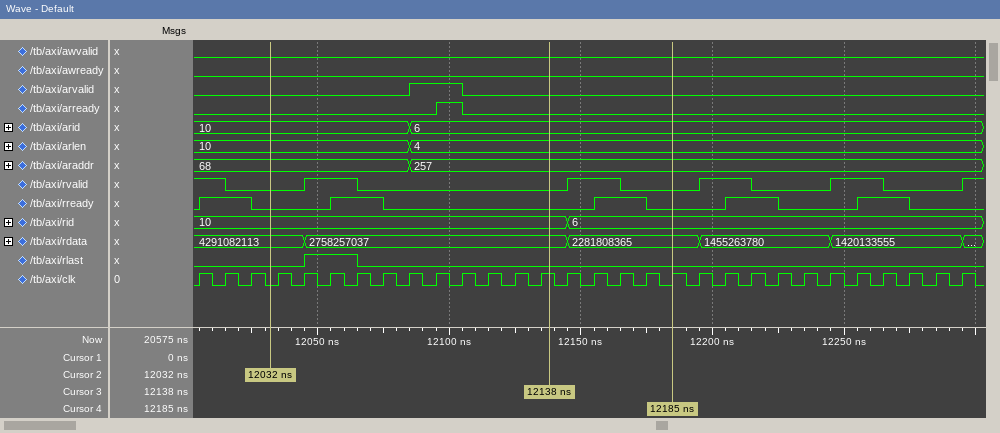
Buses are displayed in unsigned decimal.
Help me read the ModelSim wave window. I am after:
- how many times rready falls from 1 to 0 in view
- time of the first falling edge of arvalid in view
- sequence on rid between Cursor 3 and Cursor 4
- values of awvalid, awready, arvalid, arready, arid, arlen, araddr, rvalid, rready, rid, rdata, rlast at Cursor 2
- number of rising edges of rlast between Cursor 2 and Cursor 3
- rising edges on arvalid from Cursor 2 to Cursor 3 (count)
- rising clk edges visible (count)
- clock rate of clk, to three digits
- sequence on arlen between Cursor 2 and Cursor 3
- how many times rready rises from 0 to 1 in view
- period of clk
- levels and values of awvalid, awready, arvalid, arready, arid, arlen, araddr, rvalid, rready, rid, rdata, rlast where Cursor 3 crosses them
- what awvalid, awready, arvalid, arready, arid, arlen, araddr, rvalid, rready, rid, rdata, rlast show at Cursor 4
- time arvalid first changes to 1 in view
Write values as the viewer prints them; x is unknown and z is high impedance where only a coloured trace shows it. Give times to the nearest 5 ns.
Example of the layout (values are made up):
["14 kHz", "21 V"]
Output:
["5", "12105 ns", "10, 6", "awvalid=0, awready=0, arvalid=0, arready=0, arid=10, arlen=10, araddr=68, rvalid=0, rready=0, rid=10, rdata=4291082113, rlast=0", "1", "1", "30", "100 MHz", "10, 4", "5", "10 ns", "awvalid=0, awready=0, arvalid=0, arready=0, arid=6, arlen=4, araddr=257, rvalid=0, rready=0, rid=10, rdata=2758257037, rlast=0", "awvalid=0, awready=0, arvalid=0, arready=0, arid=6, arlen=4, araddr=257, rvalid=0, rready=0, rid=6, rdata=2281808365, rlast=0", "12085 ns"]
